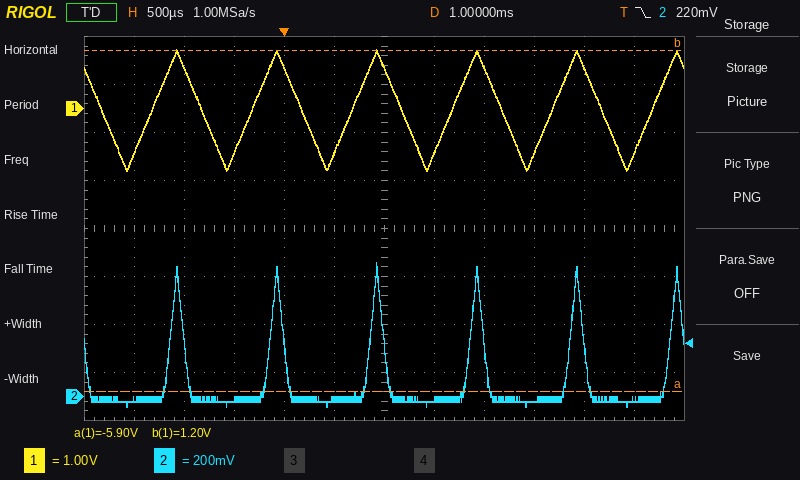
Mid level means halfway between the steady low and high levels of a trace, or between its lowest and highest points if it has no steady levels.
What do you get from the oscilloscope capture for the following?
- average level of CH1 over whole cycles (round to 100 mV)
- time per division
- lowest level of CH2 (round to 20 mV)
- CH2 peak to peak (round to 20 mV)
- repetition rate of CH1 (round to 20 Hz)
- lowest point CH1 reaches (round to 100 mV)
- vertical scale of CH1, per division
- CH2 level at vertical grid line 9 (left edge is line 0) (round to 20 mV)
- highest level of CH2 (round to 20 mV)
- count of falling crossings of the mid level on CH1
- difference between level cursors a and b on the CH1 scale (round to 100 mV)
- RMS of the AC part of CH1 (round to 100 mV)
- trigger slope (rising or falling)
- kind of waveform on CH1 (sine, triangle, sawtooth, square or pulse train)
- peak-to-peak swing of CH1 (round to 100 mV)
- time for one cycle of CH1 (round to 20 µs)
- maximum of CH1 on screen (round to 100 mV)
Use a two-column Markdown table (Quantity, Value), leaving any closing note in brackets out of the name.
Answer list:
| Quantity | Value |
|---|---|
| average level of CH1 over whole cycles | 0.0 V |
| time per division | 500 µs |
| lowest level of CH2 | -40 mV |
| CH2 peak to peak | 600 mV |
| repetition rate of CH1 | 1.00 kHz |
| lowest point CH1 reaches | -1.3 V |
| vertical scale of CH1, per division | 1 V |
| CH2 level at vertical grid line 9 (left edge is line 0) | -20 mV |
| highest level of CH2 | 560 mV |
| count of falling crossings of the mid level on CH1 | 6 |
| difference between level cursors a and b on the CH1 scale | 7.1 V |
| RMS of the AC part of CH1 | 700 mV |
| trigger slope | falling |
| kind of waveform on CH1 | triangle |
| peak-to-peak swing of CH1 | 2.5 V |
| time for one cycle of CH1 | 1.00 ms |
| maximum of CH1 on screen | 1.2 V |
